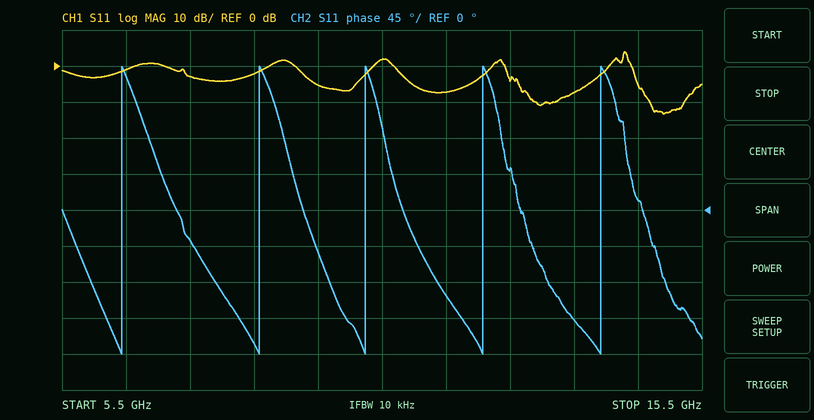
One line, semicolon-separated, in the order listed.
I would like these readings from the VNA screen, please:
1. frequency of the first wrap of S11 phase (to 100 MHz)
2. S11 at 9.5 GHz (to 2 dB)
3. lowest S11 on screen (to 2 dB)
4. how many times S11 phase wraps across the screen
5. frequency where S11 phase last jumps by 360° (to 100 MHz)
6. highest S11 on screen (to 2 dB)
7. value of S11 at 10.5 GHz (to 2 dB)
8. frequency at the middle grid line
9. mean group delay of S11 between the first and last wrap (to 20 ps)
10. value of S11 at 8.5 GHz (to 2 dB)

6.4 GHz; -6 dB; -14 dB; 5; 13.9 GHz; 4 dB; 2 dB; 10.5 GHz; 540 ps; -2 dB
